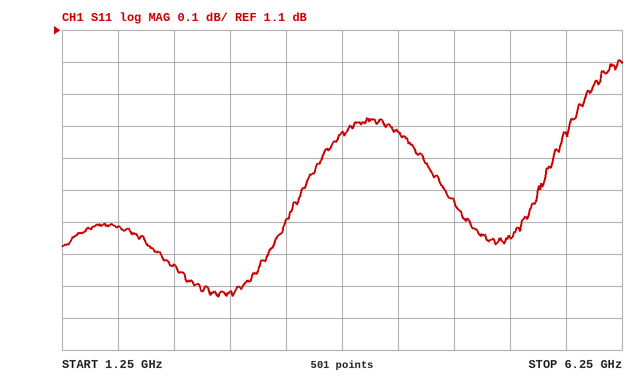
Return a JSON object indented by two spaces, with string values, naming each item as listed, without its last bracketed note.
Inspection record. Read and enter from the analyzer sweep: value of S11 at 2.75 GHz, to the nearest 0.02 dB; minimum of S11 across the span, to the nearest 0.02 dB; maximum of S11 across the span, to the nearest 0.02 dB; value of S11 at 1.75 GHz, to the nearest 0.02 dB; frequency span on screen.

{
  "value of S11 at 2.75 GHz, to the nearest 0.02 dB": "0.28 dB",
  "minimum of S11 across the span, to the nearest 0.02 dB": "0.26 dB",
  "maximum of S11 across the span, to the nearest 0.02 dB": "1.00 dB",
  "value of S11 at 1.75 GHz, to the nearest 0.02 dB": "0.48 dB",
  "frequency span on screen": "5 GHz"
}
